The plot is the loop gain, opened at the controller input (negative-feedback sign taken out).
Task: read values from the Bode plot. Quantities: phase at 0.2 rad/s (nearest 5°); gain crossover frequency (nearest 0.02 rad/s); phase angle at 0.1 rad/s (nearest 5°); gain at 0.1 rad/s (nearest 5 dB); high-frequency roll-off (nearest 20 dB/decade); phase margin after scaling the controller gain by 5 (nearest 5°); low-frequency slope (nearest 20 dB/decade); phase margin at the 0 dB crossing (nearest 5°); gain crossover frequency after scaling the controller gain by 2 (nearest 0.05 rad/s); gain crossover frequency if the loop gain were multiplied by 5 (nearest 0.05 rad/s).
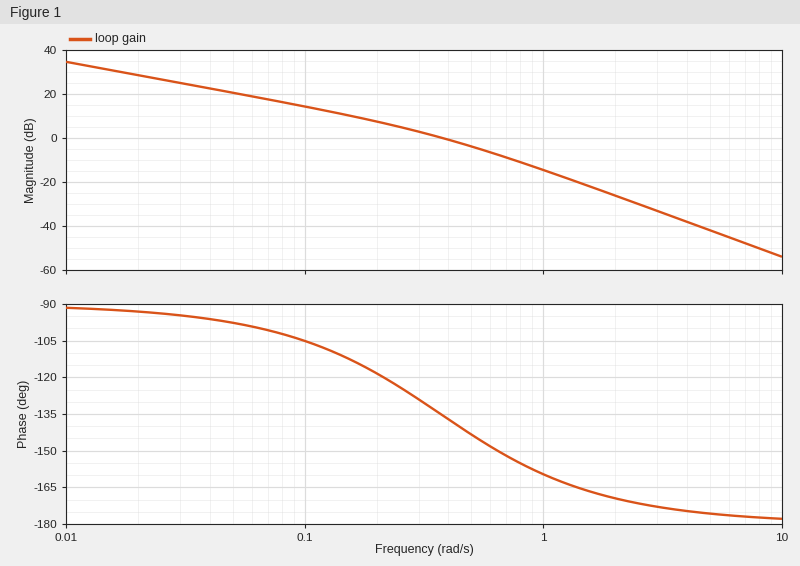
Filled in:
-120°
0.38 rad/s
-105°
15 dB
-40 dB/decade
20°
-20 dB/decade
45°
0.60 rad/s
0.95 rad/s
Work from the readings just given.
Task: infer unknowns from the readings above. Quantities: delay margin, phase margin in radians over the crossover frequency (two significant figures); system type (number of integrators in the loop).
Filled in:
2.1 s
1
